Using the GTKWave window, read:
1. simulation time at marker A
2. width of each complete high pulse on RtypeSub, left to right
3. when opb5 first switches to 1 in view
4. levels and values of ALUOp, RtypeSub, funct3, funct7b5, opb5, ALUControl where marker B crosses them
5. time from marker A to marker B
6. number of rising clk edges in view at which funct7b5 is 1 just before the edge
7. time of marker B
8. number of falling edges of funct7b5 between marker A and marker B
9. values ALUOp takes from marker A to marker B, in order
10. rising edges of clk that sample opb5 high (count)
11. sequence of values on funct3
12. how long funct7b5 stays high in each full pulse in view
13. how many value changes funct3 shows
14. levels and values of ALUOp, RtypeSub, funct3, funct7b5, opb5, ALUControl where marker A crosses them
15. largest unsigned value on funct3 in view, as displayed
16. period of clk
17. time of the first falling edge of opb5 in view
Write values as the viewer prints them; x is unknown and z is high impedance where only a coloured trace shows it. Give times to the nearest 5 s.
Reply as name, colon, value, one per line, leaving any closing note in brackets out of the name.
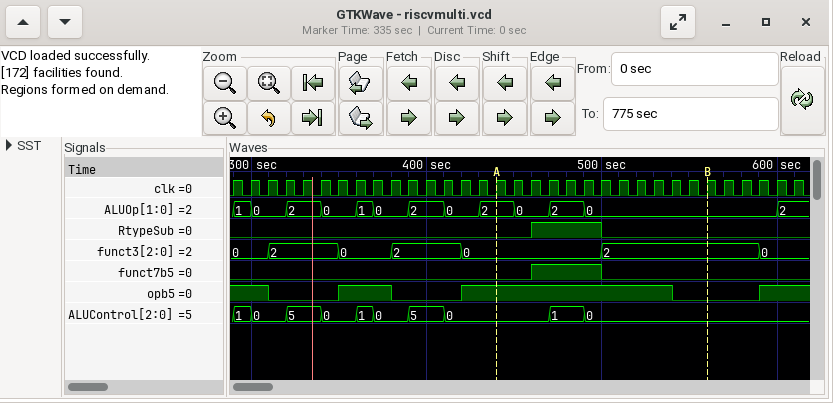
simulation time at marker A: 440 s
width of each complete high pulse on RtypeSub, left to right: 40 s
when opb5 first switches to 1 in view: 350 s
levels and values of ALUOp, RtypeSub, funct3, funct7b5, opb5, ALUControl where marker B crosses them: ALUOp=0, RtypeSub=0, funct3=2, funct7b5=0, opb5=0, ALUControl=0
time from marker A to marker B: 120 s
number of rising clk edges in view at which funct7b5 is 1 just before the edge: 4
time of marker B: 560 s
number of falling edges of funct7b5 between marker A and marker B: 1
values ALUOp takes from marker A to marker B, in order: 2, 0, 2, 0
rising edges of clk that sample opb5 high: 20
sequence of values on funct3: 0, 2, 0, 2, 0, 2, 0
how long funct7b5 stays high in each full pulse in view: 40 s
how many value changes funct3 shows: 6
levels and values of ALUOp, RtypeSub, funct3, funct7b5, opb5, ALUControl where marker A crosses them: ALUOp=2, RtypeSub=0, funct3=0, funct7b5=0, opb5=1, ALUControl=0
largest unsigned value on funct3 in view, as displayed: 2
period of clk: 10 s
time of the first falling edge of opb5 in view: 310 s
